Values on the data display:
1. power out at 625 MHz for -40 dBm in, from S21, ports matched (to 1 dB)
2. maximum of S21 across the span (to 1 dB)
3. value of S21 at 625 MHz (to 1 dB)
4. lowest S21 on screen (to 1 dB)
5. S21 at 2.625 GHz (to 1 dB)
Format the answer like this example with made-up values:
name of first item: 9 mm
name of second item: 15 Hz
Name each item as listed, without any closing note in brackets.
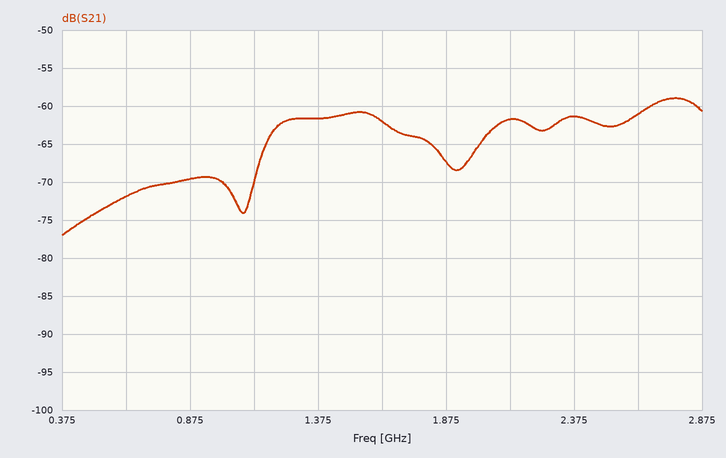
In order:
power out at 625 MHz for -40 dBm in, from S21, ports matched: -112 dBm
maximum of S21 across the span: -59 dB
value of S21 at 625 MHz: -72 dB
lowest S21 on screen: -77 dB
S21 at 2.625 GHz: -61 dB
